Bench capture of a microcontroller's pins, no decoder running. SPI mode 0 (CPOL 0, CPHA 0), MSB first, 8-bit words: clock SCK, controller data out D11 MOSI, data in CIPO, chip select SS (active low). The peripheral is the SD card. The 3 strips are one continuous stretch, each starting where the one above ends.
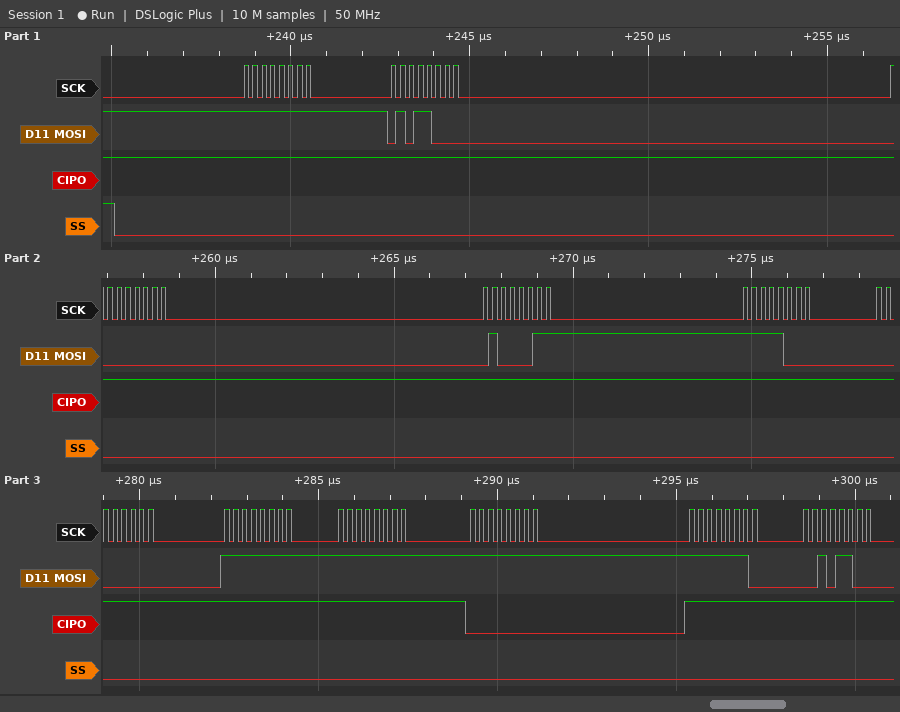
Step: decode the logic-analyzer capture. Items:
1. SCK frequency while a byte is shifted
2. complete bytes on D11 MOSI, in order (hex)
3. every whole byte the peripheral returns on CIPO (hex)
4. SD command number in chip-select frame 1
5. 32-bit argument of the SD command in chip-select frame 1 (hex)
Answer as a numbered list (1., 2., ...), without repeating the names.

1. 4 MHz
2. FF 58 00 43 F8 00 FF FF FF FE 2C
3. FF FF FF FF FF FF FF FF 00 FF FF
4. CMD24
5. 0x0043F800
